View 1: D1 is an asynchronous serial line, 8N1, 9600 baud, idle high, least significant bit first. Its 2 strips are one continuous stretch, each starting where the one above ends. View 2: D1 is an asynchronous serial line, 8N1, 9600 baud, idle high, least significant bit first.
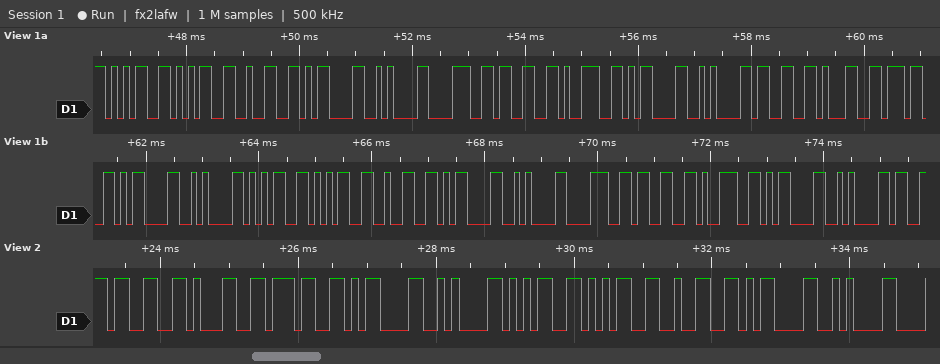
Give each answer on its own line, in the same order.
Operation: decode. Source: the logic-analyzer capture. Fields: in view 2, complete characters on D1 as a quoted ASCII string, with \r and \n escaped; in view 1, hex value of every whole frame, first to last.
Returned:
"317\r\n552\r\n"
35 35 32 0D 0A 38 33 39 0D 0A 33 31 37 0D 0A 35 35 32 0D 0A 38 33 39 0D 0A
